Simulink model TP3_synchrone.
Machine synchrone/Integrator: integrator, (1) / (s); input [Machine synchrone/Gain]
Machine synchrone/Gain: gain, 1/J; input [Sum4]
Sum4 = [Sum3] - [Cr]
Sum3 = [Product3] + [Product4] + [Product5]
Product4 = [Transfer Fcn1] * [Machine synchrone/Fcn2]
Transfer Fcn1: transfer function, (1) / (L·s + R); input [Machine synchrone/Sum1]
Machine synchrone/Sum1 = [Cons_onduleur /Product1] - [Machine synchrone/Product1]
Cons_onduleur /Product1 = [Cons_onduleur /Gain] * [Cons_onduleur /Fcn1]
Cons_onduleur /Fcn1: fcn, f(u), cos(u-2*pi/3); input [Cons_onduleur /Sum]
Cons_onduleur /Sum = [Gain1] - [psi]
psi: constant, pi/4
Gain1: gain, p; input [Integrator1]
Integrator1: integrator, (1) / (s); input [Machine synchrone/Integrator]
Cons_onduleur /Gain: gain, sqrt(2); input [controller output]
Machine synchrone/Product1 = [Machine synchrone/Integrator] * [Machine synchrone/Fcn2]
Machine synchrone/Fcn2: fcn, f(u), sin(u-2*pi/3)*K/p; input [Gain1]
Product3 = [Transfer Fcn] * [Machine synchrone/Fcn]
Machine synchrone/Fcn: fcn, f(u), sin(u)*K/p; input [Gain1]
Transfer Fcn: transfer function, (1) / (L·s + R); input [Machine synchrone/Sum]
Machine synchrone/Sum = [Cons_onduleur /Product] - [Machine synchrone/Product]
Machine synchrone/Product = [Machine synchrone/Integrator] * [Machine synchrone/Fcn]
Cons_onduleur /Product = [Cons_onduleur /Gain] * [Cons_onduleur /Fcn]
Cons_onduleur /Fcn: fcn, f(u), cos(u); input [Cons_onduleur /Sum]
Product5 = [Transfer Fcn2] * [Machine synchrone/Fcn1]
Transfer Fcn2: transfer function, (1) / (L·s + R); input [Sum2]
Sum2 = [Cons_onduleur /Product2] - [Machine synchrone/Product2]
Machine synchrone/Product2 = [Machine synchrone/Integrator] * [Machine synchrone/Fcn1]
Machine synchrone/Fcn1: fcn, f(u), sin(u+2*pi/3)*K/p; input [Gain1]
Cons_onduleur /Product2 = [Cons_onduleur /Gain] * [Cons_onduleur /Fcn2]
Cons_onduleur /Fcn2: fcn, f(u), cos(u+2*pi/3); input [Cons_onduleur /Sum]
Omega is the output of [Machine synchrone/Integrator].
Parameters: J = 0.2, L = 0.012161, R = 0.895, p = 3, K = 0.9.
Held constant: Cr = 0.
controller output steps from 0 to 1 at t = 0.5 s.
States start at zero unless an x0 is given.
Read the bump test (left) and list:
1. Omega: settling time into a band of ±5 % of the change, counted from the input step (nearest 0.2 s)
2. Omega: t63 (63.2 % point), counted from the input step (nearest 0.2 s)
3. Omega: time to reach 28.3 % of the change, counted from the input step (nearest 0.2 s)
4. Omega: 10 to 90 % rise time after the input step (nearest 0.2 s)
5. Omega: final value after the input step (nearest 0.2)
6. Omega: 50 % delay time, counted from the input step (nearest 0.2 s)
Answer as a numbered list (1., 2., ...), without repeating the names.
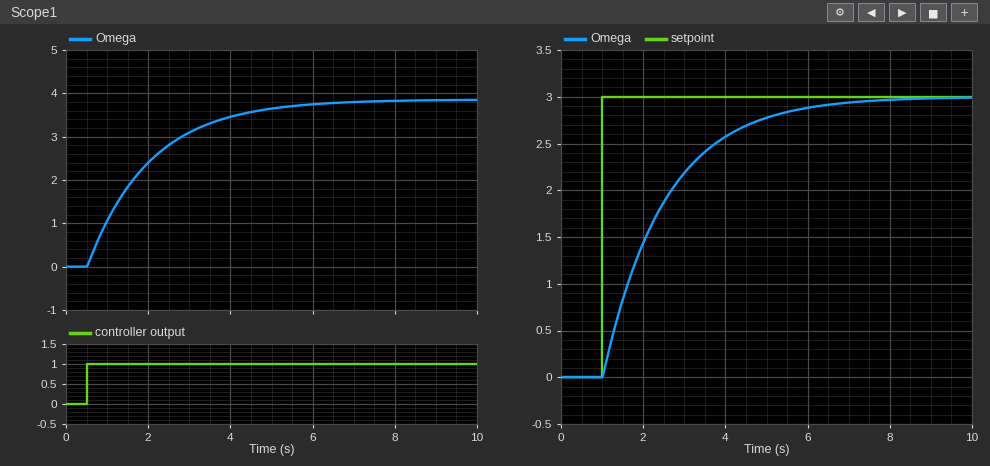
1. 4.6 s
2. 1.6 s
3. 0.6 s
4. 3.4 s
5. 3.8
6. 1.0 s
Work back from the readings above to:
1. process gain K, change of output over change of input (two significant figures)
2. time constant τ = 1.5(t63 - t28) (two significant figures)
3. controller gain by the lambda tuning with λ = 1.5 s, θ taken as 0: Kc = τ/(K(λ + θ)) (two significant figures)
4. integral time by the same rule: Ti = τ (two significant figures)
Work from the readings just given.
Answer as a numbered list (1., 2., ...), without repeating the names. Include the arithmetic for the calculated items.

1. (3.8 - 0) / 1 = 3.8
2. 1.5 × (1.6 - 0.6) = 1.5 s
3. 1.5 / (3.8 × (1.5 + 0)) = 0.26
4. 1.5 s
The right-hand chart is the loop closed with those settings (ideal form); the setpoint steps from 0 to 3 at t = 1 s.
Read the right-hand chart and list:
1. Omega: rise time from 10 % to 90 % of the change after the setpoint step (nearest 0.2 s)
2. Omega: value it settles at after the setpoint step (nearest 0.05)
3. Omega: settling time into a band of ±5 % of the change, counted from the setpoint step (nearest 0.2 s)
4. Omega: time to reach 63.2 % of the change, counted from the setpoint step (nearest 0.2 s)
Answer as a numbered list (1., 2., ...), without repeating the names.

1. 3.4 s
2. 3.00
3. 4.6 s
4. 1.6 s
